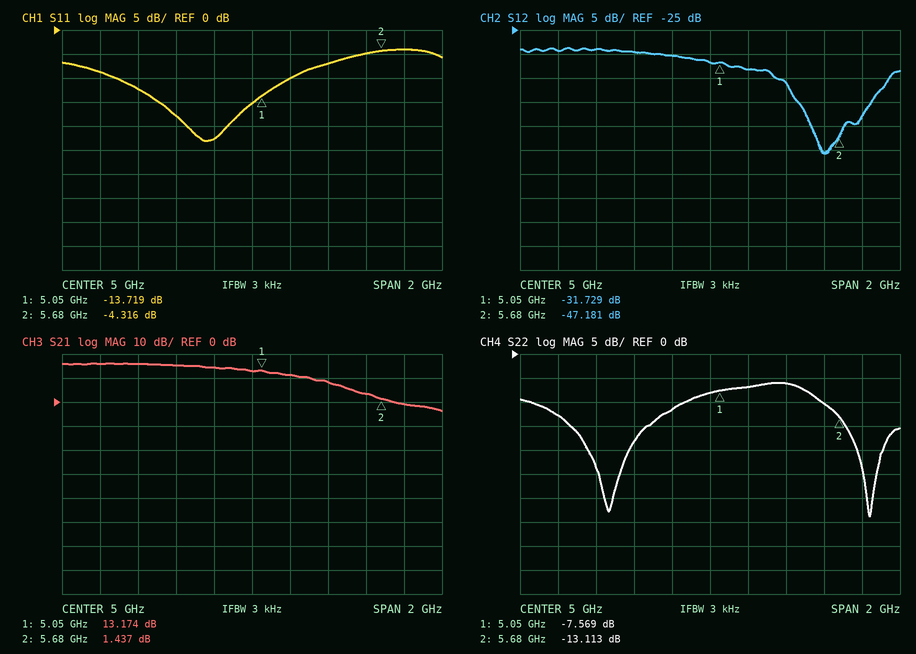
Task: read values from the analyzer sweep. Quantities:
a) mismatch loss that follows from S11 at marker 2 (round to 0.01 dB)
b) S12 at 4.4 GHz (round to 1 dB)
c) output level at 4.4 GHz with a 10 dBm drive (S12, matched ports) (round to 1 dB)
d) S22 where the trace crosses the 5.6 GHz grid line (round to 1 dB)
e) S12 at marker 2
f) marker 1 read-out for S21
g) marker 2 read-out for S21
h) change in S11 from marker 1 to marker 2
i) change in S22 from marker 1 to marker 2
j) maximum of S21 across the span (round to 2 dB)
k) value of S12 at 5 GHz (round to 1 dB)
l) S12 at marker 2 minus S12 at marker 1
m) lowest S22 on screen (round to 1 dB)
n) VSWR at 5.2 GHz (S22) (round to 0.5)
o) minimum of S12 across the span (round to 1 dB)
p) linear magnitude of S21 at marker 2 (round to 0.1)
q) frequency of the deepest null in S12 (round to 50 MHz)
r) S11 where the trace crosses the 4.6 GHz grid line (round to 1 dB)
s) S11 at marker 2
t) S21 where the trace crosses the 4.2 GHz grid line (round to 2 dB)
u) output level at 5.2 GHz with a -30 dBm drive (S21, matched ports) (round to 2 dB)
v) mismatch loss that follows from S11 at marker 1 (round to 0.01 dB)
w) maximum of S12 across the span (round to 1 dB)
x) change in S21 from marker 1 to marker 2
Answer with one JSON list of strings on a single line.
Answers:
["2.01 dB", "-29 dB", "-19 dBm", "-10 dB", "-47.181 dB", "13.174 dB", "1.437 dB", "9.403 dB", "-5.544 dB", "16 dB", "-32 dB", "-15.452 dB", "-34 dB", "2.5", "-51 dB", "1.2", "5.60 GHz", "-18 dB", "-4.316 dB", "16 dB", "-18 dBm", "0.19 dB", "-29 dB", "-11.737 dB"]
